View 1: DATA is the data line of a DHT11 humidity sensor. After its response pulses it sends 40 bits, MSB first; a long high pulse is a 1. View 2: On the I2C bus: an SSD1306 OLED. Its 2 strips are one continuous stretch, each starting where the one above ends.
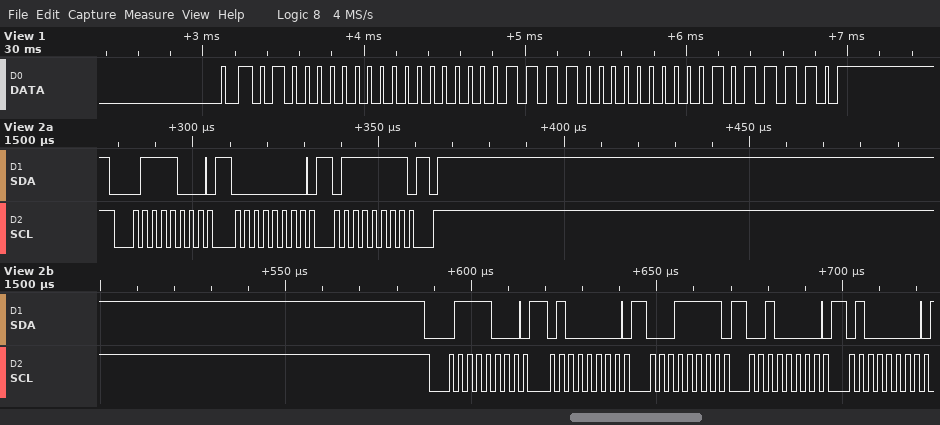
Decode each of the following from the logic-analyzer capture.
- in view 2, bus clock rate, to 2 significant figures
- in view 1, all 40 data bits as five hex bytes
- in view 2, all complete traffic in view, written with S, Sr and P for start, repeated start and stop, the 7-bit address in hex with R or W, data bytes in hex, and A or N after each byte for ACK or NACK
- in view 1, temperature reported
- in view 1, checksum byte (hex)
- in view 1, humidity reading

400 kHz
40 00 1E 00 5E
S 3CW A 00 A 7F A P S 3CW A 40 A 1F A 20 A 40 A
30.0 °C
0x5E
64 %
